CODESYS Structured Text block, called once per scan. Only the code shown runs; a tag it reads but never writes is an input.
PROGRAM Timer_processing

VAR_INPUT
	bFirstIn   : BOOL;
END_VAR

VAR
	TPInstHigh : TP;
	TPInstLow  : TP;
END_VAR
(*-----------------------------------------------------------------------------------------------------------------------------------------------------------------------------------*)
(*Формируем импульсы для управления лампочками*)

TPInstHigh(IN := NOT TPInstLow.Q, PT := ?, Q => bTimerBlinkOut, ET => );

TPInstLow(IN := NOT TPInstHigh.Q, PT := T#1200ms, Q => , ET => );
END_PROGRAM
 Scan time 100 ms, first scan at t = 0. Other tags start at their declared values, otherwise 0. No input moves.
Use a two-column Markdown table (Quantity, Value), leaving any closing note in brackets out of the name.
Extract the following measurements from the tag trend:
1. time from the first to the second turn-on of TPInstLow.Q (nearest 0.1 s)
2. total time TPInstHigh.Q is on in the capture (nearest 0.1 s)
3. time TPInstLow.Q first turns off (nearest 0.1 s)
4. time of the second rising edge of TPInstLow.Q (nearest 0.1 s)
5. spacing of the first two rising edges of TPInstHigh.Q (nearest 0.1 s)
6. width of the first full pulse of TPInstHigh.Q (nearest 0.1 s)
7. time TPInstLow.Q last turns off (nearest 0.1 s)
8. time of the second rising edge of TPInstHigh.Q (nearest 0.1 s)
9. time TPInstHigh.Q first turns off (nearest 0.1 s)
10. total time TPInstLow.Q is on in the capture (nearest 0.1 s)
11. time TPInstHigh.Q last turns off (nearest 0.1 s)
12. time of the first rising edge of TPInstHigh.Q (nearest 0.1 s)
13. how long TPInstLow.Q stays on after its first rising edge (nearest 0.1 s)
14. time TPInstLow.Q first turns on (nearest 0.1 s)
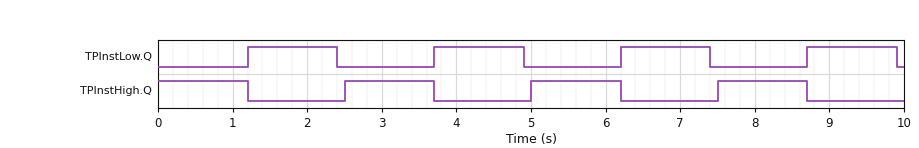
| Quantity | Value |
|---|---|
| time from the first to the second turn-on of TPInstLow.Q | 2.5 s |
| total time TPInstHigh.Q is on in the capture | 4.8 s |
| time TPInstLow.Q first turns off | 2.4 s |
| time of the second rising edge of TPInstLow.Q | 3.7 s |
| spacing of the first two rising edges of TPInstHigh.Q | 2.5 s |
| width of the first full pulse of TPInstHigh.Q | 1.2 s |
| time TPInstLow.Q last turns off | 9.9 s |
| time of the second rising edge of TPInstHigh.Q | 5.0 s |
| time TPInstHigh.Q first turns off | 1.2 s |
| total time TPInstLow.Q is on in the capture | 4.8 s |
| time TPInstHigh.Q last turns off | 8.7 s |
| time of the first rising edge of TPInstHigh.Q | 2.5 s |
| how long TPInstLow.Q stays on after its first rising edge | 1.2 s |
| time TPInstLow.Q first turns on | 1.2 s |
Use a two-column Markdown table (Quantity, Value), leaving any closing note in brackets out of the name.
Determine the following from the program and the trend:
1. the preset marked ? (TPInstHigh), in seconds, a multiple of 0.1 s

| Quantity | Value |
|---|---|
| the preset marked ? (TPInstHigh), in seconds, a multiple of 0.1 s | 1.2 s |
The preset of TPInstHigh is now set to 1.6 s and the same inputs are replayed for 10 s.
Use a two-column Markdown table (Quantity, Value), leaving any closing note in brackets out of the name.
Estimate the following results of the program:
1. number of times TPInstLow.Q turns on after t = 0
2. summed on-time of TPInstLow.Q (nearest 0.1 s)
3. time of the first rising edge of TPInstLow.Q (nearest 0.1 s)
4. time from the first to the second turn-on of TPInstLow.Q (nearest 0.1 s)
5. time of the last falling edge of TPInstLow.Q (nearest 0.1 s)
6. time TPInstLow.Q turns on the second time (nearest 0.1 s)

| Quantity | Value |
|---|---|
| number of times TPInstLow.Q turns on after t = 0 | 3 |
| summed on-time of TPInstLow.Q | 3.6 s |
| time of the first rising edge of TPInstLow.Q | 1.6 s |
| time from the first to the second turn-on of TPInstLow.Q | 2.9 s |
| time of the last falling edge of TPInstLow.Q | 8.6 s |
| time TPInstLow.Q turns on the second time | 4.5 s |
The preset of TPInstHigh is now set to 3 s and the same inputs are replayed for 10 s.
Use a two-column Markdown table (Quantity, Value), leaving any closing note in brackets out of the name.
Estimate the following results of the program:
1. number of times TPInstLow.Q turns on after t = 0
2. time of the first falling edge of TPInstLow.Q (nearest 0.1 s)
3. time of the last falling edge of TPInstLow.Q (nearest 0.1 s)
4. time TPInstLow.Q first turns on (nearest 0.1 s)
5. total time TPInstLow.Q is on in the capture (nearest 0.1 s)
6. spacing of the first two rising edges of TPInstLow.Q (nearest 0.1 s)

| Quantity | Value |
|---|---|
| number of times TPInstLow.Q turns on after t = 0 | 2 |
| time of the first falling edge of TPInstLow.Q | 4.2 s |
| time of the last falling edge of TPInstLow.Q | 8.5 s |
| time TPInstLow.Q first turns on | 3.0 s |
| total time TPInstLow.Q is on in the capture | 2.4 s |
| spacing of the first two rising edges of TPInstLow.Q | 4.3 s |
